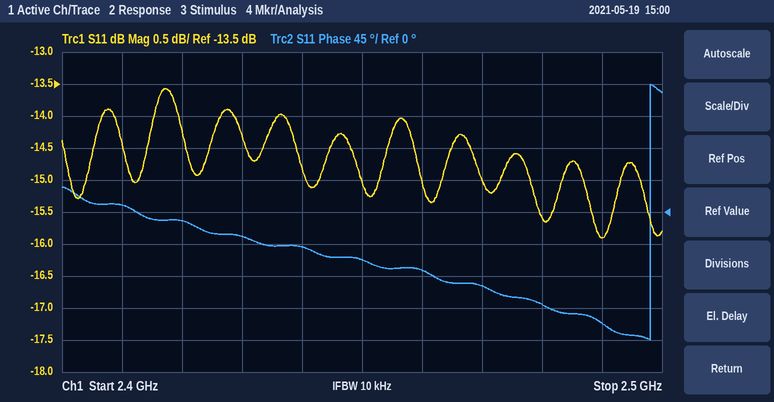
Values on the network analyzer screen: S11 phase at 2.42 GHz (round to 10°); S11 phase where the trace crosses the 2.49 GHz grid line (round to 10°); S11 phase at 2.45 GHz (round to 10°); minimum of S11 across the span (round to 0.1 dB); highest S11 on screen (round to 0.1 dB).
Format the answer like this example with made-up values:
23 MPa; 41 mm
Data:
-10°; -160°; -70°; -15.9 dB; -13.6 dB
